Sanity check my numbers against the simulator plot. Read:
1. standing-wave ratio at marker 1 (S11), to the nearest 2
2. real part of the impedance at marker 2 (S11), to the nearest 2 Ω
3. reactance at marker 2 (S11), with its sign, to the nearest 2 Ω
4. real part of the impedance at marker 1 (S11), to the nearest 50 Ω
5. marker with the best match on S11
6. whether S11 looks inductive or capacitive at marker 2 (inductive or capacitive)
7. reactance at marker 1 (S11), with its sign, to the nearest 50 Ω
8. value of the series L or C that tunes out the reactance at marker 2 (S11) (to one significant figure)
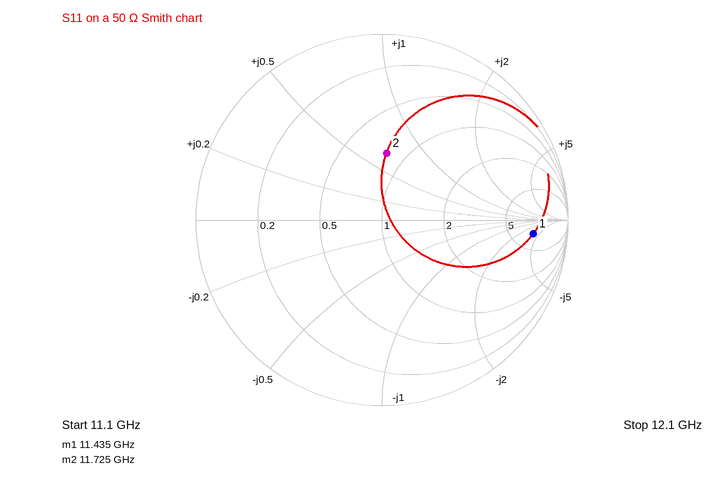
10
40 Ω
+34 Ω
400 Ω
marker 2
inductive
-200 Ω
400 fF
